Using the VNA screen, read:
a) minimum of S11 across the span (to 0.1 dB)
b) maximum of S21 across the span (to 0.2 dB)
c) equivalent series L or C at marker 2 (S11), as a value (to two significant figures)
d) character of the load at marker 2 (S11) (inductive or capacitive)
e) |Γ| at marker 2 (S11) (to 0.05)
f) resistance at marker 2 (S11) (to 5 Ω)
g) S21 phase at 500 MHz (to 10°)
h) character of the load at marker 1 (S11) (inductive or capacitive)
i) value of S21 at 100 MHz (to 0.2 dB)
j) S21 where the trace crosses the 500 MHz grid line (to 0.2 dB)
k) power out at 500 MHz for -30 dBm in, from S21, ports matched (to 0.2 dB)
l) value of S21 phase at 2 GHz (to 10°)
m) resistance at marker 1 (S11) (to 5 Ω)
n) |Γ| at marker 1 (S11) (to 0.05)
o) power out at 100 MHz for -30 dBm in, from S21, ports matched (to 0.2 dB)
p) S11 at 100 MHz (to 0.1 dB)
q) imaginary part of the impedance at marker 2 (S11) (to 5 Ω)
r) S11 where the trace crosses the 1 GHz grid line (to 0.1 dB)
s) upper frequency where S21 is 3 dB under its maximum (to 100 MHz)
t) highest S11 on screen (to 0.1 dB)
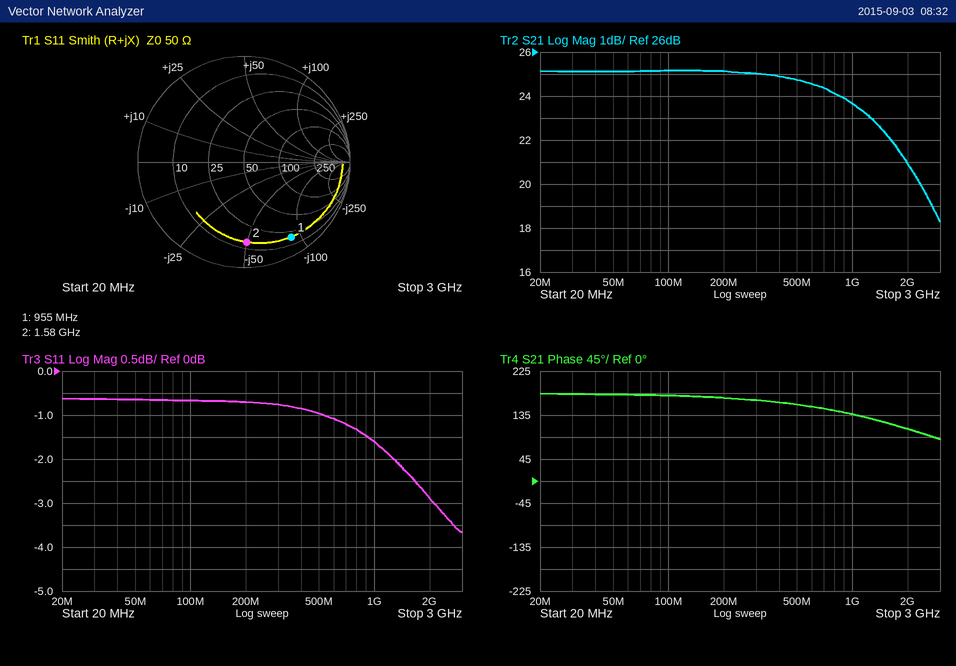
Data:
-3.7 dB
25.2 dB
2.0 pF
capacitive
0.75
15 Ω
160°
capacitive
25.2 dB
24.8 dB
-5.2 dBm
110°
20 Ω
0.85
-4.8 dBm
-0.7 dB
-50 Ω
-1.6 dB
1.6 GHz
-0.6 dB
